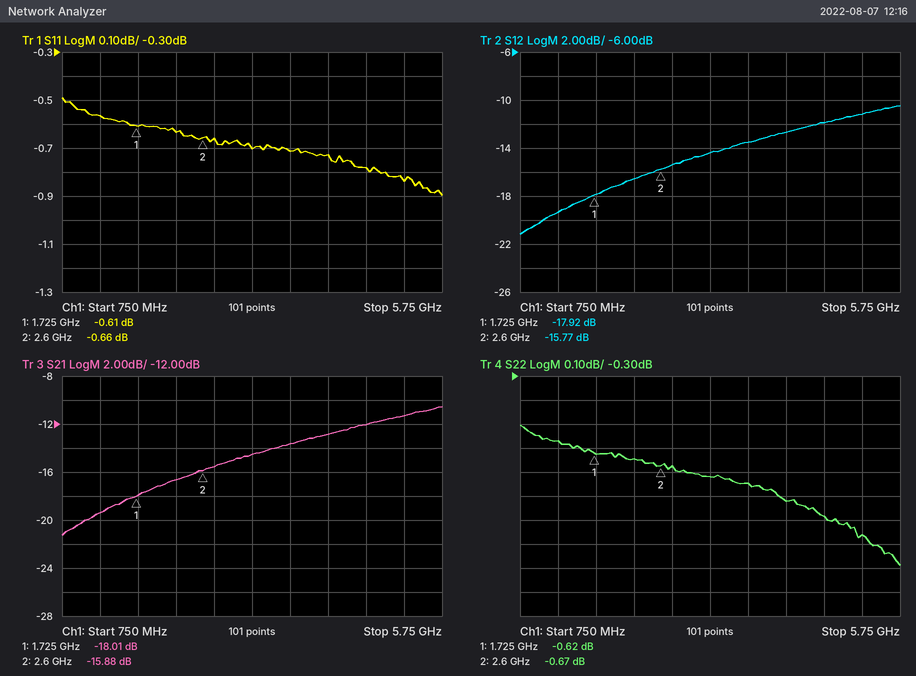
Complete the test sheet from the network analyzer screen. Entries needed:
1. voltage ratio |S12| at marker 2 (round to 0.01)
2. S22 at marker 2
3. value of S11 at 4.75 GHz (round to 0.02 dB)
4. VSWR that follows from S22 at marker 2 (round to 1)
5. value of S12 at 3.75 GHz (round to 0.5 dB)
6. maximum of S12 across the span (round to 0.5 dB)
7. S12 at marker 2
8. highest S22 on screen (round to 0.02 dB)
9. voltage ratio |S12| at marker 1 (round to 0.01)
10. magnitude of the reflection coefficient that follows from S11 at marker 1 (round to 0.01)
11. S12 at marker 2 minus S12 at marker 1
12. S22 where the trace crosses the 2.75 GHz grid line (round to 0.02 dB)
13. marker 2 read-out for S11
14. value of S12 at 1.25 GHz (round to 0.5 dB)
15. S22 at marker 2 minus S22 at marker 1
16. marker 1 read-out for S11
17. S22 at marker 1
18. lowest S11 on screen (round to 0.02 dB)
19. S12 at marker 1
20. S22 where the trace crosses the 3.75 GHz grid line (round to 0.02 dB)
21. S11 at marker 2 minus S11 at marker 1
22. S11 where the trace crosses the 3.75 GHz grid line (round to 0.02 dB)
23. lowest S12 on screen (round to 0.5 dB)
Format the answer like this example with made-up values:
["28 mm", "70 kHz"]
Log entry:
["0.16", "-0.67 dB", "-0.78 dB", "26", "-13.5 dB", "-10.5 dB", "-15.77 dB", "-0.50 dB", "0.13", "0.93", "2.15 dB", "-0.68 dB", "-0.66 dB", "-19.5 dB", "-0.05 dB", "-0.61 dB", "-0.62 dB", "-0.90 dB", "-17.92 dB", "-0.74 dB", "-0.05 dB", "-0.72 dB", "-21.0 dB"]
